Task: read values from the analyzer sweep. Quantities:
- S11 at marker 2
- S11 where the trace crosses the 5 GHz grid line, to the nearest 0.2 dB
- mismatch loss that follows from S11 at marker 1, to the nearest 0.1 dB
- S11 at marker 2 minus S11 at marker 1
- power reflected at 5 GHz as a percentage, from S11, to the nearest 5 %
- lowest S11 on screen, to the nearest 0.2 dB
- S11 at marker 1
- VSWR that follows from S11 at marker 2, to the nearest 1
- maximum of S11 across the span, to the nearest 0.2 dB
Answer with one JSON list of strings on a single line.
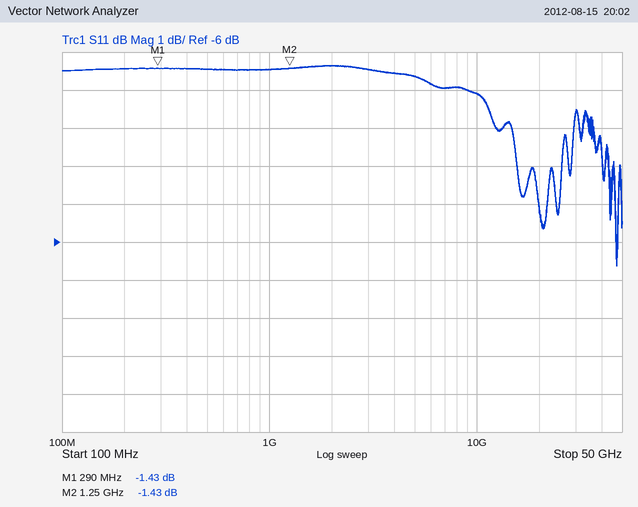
["-1.43 dB", "-1.6 dB", "5.5 dB", "0.00 dB", "70 %", "-6.6 dB", "-1.43 dB", "12", "-1.4 dB"]
